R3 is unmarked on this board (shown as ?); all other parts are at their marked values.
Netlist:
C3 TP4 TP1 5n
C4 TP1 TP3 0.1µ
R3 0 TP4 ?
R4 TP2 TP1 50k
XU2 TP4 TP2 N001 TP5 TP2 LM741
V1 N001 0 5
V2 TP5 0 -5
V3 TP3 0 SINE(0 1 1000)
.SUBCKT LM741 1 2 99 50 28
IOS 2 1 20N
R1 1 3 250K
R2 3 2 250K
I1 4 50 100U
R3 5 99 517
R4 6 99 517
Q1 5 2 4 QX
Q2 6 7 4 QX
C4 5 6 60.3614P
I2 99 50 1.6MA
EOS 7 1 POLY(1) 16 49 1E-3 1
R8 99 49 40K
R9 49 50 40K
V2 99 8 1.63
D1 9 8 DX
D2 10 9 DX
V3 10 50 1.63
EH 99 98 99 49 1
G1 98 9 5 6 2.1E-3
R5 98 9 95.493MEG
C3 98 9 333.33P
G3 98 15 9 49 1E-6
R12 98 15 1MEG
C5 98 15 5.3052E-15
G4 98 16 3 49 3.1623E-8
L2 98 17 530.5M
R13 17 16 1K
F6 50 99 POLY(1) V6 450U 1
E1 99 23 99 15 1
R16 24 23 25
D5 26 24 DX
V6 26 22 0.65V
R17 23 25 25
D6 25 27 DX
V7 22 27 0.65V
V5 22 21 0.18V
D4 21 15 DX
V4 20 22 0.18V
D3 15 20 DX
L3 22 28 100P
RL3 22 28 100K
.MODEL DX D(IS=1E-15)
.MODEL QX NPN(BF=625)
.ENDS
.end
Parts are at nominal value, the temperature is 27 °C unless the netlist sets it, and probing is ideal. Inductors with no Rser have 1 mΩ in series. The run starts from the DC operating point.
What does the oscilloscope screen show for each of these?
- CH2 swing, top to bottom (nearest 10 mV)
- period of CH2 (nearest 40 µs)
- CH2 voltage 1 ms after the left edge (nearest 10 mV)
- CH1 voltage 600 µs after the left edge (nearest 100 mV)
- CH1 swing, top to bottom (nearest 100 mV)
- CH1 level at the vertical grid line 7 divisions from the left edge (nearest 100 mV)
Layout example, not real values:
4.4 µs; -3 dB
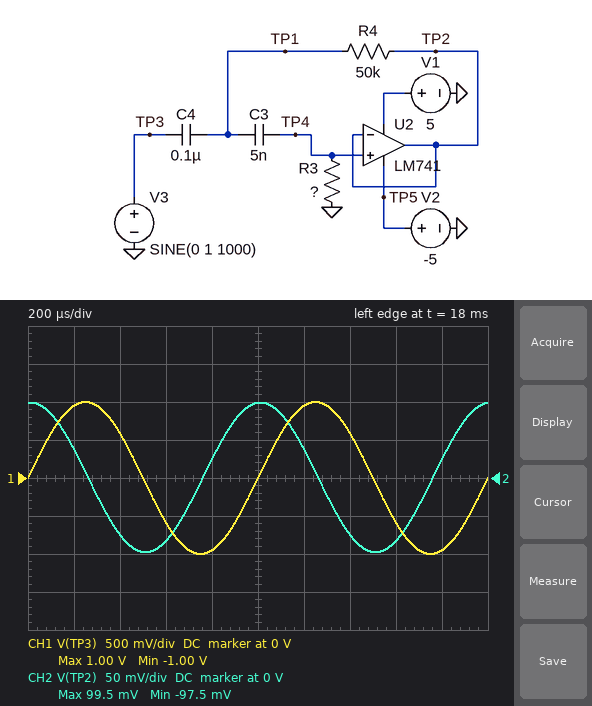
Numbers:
200 mV; 1.00 ms; 100 mV; -600 mV; 2.0 V; 600 mV
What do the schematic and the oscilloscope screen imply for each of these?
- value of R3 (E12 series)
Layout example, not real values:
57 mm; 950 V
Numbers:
3.3 kΩ
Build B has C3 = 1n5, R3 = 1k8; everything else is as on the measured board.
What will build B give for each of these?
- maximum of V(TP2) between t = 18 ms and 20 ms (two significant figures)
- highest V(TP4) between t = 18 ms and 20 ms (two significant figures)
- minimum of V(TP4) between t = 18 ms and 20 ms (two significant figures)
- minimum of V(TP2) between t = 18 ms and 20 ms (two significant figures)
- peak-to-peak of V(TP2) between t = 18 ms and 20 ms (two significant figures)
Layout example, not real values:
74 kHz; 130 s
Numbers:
18 mV; 17 mV; -17 mV; -16 mV; 33 mV
